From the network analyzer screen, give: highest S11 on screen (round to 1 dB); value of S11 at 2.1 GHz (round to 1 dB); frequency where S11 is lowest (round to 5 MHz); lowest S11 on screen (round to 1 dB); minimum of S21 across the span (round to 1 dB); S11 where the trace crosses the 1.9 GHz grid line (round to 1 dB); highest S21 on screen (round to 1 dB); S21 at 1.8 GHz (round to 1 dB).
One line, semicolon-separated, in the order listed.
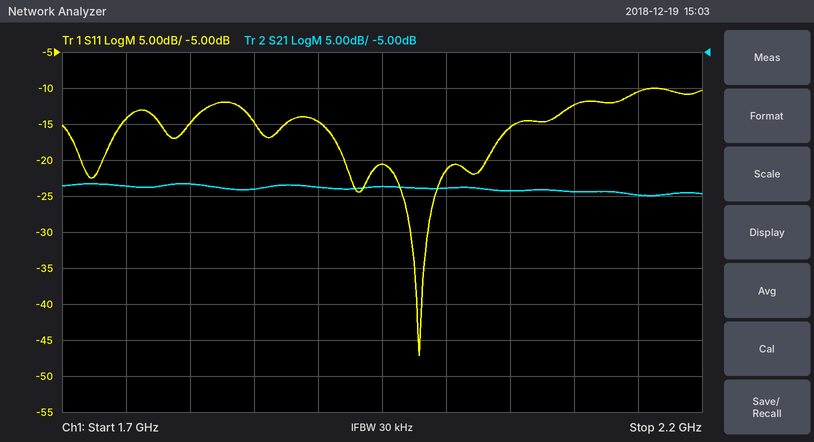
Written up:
-10 dB; -12 dB; 1.980 GHz; -47 dB; -25 dB; -15 dB; -23 dB; -23 dB
